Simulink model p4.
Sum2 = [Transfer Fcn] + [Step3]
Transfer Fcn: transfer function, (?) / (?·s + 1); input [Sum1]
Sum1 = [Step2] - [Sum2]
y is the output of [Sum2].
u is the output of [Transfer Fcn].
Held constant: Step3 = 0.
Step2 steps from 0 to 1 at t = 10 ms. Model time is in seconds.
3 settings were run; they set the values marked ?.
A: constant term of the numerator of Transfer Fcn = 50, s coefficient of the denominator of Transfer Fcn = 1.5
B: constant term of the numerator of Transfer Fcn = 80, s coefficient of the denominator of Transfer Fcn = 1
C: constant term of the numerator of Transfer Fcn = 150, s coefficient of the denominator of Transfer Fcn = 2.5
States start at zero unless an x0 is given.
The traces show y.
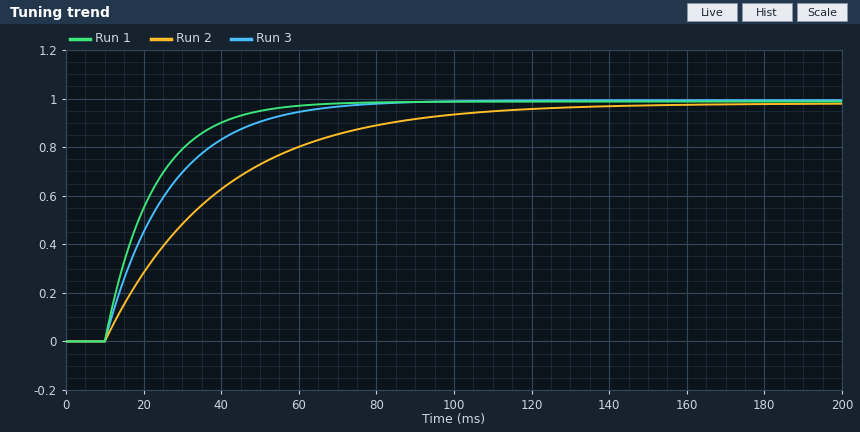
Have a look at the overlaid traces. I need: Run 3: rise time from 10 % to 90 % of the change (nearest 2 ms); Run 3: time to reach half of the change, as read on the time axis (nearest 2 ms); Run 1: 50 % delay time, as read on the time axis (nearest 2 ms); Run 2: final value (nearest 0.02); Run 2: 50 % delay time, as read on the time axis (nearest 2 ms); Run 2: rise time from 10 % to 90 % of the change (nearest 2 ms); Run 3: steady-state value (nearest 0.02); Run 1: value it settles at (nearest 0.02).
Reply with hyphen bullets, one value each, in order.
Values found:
- 36 ms
- 22 ms
- 18 ms
- 0.98
- 30 ms
- 64 ms
- 1.00
- 0.98
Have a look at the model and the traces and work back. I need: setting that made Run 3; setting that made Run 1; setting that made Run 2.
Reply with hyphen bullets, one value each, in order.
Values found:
- C
- B
- A
